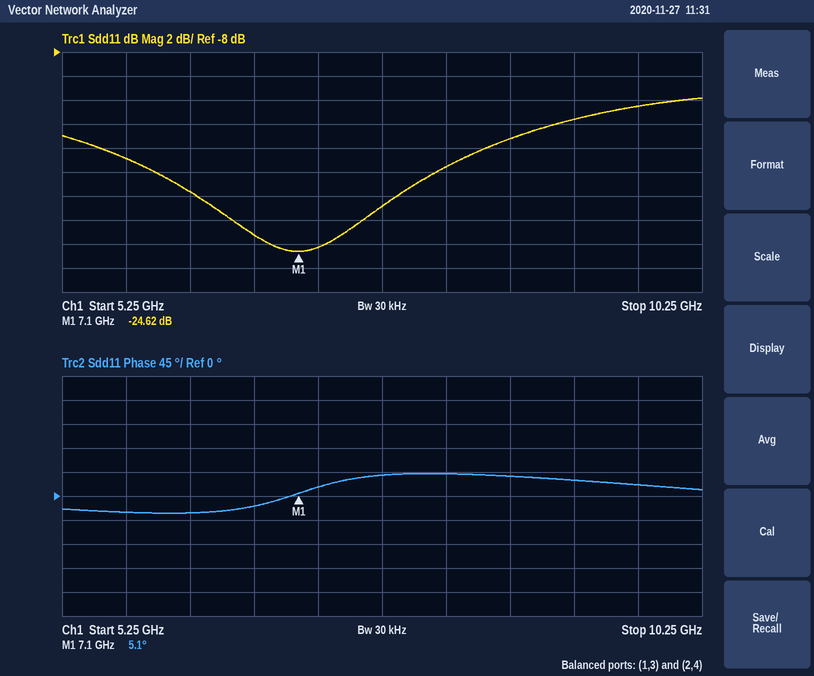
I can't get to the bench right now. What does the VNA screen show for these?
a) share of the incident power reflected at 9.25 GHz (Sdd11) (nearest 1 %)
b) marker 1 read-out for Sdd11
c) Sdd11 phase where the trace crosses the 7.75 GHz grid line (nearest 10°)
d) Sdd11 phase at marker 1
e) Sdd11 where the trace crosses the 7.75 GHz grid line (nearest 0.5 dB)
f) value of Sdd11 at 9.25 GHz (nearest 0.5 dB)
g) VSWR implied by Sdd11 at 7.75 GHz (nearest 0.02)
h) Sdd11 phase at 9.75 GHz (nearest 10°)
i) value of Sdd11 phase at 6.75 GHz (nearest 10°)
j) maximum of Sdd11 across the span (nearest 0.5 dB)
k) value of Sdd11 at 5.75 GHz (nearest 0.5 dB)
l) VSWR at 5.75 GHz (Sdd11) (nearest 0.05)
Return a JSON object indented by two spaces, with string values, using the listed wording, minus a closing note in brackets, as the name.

{
  "share of the incident power reflected at 9.25 GHz (Sdd11)": "4 %",
  "marker 1 read-out for Sdd11": "-24.62 dB",
  "Sdd11 phase where the trace crosses the 7.75 GHz grid line": "40°",
  "Sdd11 phase at marker 1": "5.1°",
  "Sdd11 where the trace crosses the 7.75 GHz grid line": "-21.0 dB",
  "value of Sdd11 at 9.25 GHz": "-13.5 dB",
  "VSWR implied by Sdd11 at 7.75 GHz": "1.20",
  "Sdd11 phase at 9.75 GHz": "20°",
  "value of Sdd11 phase at 6.75 GHz": "-20°",
  "maximum of Sdd11 across the span": "-12.0 dB",
  "value of Sdd11 at 5.75 GHz": "-17.0 dB",
  "VSWR at 5.75 GHz (Sdd11)": "1.35"
}
